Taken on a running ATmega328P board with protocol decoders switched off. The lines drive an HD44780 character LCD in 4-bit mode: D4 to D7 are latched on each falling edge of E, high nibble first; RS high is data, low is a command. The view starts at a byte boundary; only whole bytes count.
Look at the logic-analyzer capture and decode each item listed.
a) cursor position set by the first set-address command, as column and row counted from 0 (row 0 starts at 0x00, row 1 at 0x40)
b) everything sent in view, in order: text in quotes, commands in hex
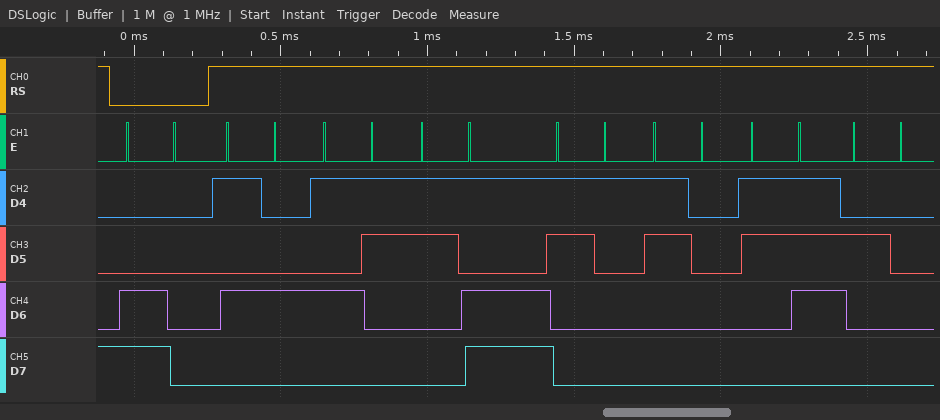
column 0, row 1
0xC0 "TS=107 "
